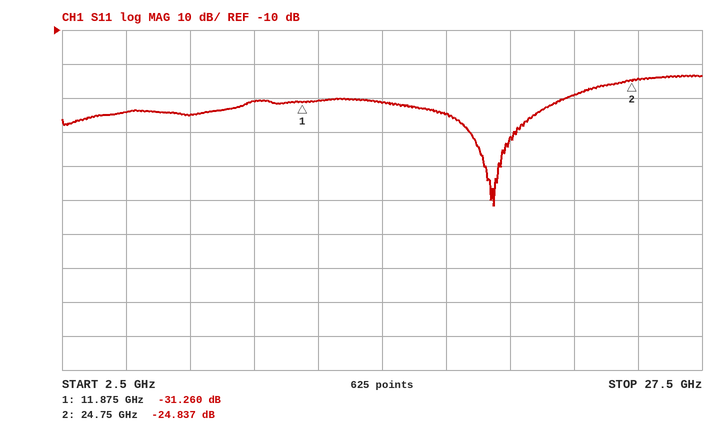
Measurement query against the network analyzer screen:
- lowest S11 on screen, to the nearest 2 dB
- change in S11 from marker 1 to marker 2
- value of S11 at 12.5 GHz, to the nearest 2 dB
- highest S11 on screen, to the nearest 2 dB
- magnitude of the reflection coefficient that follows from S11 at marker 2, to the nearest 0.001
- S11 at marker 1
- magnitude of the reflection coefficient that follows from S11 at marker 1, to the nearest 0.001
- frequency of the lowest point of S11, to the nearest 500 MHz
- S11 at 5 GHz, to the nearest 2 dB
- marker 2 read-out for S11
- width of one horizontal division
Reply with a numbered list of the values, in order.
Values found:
1. -62 dB
2. 6.423 dB
3. -30 dB
4. -24 dB
5. 0.057
6. -31.260 dB
7. 0.027
8. 19.5 GHz
9. -34 dB
10. -24.837 dB
11. 2.5 GHz
